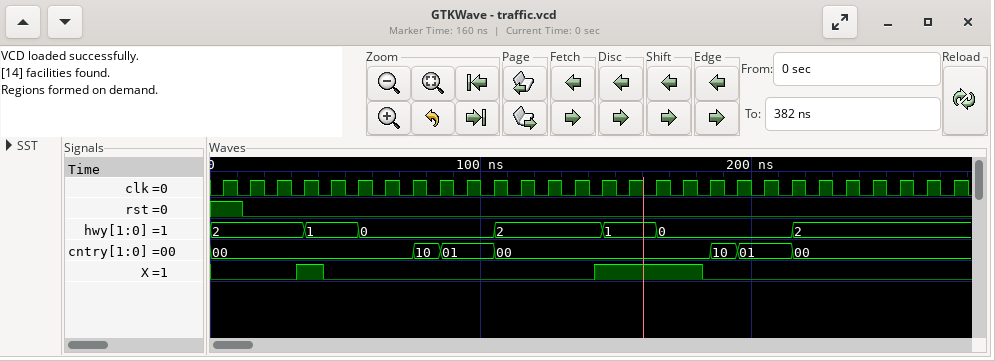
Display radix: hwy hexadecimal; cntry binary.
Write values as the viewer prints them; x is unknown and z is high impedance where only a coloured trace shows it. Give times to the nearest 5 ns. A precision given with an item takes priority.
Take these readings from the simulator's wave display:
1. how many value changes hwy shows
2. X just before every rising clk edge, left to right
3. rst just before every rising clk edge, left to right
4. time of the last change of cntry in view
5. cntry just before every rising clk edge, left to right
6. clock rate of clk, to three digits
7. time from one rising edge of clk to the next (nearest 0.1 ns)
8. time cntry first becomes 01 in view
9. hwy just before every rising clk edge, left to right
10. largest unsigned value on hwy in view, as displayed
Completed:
6
0 0 0 1 0 0 0 0 0 0 0 0 0 0 1 1 1 1 0 0 0 0 0 0 0 0 0 0
1 0 0 0 0 0 0 0 0 0 0 0 0 0 0 0 0 0 0 0 0 0 0 0 0 0 0 0
215 ns
00, 00, 00, 00, 00, 00, 00, 00, 10, 01, 01, 00, 00, 00, 00, 00, 00, 00, 00, 10, 01, 01, 00, 00, 00, 00, 00, 00
100 MHz
10 ns
85 ns
2, 2, 2, 2, 1, 1, 0, 0, 0, 0, 0, 2, 2, 2, 2, 1, 1, 0, 0, 0, 0, 0, 2, 2, 2, 2, 2, 2
2
